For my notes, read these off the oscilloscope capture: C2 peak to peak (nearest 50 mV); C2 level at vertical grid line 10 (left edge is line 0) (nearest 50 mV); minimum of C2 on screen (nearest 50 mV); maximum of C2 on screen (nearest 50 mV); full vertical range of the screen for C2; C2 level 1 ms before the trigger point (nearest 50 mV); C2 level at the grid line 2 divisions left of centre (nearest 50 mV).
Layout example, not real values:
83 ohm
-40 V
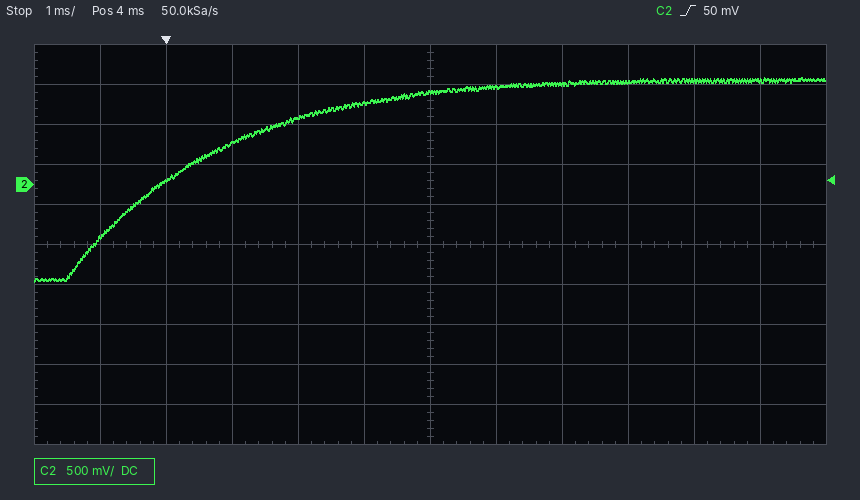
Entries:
2.55 V
1.30 V
-1.20 V
1.35 V
5 V
-650 mV
850 mV
